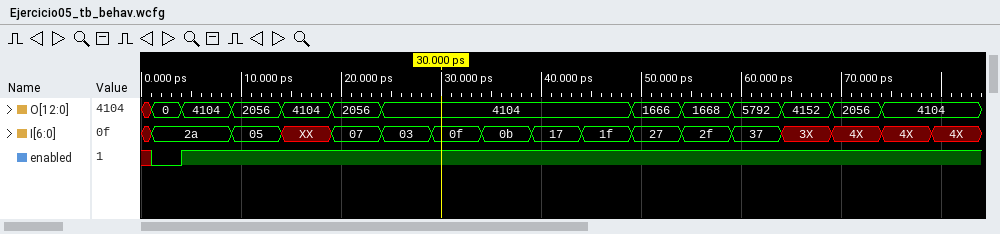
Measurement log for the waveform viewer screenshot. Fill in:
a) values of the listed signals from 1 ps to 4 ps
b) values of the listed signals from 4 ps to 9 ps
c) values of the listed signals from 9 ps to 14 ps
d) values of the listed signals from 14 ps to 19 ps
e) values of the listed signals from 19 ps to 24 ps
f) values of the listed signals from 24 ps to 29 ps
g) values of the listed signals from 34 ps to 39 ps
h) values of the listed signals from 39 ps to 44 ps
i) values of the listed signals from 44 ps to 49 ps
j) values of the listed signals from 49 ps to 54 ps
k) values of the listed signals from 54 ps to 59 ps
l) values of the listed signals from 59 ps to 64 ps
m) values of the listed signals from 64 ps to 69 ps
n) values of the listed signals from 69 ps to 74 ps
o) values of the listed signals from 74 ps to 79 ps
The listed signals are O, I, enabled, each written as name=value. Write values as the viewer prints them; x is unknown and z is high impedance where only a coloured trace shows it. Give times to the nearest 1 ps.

O=0, I=2a, enabled=0
O=4104, I=2a, enabled=1
O=2056, I=05, enabled=1
O=4104, I=XX, enabled=1
O=2056, I=07, enabled=1
O=4104, I=03, enabled=1
O=4104, I=0b, enabled=1
O=4104, I=17, enabled=1
O=4104, I=1f, enabled=1
O=1666, I=27, enabled=1
O=1668, I=2f, enabled=1
O=5792, I=37, enabled=1
O=4152, I=3X, enabled=1
O=2056, I=4X, enabled=1
O=4104, I=4X, enabled=1
